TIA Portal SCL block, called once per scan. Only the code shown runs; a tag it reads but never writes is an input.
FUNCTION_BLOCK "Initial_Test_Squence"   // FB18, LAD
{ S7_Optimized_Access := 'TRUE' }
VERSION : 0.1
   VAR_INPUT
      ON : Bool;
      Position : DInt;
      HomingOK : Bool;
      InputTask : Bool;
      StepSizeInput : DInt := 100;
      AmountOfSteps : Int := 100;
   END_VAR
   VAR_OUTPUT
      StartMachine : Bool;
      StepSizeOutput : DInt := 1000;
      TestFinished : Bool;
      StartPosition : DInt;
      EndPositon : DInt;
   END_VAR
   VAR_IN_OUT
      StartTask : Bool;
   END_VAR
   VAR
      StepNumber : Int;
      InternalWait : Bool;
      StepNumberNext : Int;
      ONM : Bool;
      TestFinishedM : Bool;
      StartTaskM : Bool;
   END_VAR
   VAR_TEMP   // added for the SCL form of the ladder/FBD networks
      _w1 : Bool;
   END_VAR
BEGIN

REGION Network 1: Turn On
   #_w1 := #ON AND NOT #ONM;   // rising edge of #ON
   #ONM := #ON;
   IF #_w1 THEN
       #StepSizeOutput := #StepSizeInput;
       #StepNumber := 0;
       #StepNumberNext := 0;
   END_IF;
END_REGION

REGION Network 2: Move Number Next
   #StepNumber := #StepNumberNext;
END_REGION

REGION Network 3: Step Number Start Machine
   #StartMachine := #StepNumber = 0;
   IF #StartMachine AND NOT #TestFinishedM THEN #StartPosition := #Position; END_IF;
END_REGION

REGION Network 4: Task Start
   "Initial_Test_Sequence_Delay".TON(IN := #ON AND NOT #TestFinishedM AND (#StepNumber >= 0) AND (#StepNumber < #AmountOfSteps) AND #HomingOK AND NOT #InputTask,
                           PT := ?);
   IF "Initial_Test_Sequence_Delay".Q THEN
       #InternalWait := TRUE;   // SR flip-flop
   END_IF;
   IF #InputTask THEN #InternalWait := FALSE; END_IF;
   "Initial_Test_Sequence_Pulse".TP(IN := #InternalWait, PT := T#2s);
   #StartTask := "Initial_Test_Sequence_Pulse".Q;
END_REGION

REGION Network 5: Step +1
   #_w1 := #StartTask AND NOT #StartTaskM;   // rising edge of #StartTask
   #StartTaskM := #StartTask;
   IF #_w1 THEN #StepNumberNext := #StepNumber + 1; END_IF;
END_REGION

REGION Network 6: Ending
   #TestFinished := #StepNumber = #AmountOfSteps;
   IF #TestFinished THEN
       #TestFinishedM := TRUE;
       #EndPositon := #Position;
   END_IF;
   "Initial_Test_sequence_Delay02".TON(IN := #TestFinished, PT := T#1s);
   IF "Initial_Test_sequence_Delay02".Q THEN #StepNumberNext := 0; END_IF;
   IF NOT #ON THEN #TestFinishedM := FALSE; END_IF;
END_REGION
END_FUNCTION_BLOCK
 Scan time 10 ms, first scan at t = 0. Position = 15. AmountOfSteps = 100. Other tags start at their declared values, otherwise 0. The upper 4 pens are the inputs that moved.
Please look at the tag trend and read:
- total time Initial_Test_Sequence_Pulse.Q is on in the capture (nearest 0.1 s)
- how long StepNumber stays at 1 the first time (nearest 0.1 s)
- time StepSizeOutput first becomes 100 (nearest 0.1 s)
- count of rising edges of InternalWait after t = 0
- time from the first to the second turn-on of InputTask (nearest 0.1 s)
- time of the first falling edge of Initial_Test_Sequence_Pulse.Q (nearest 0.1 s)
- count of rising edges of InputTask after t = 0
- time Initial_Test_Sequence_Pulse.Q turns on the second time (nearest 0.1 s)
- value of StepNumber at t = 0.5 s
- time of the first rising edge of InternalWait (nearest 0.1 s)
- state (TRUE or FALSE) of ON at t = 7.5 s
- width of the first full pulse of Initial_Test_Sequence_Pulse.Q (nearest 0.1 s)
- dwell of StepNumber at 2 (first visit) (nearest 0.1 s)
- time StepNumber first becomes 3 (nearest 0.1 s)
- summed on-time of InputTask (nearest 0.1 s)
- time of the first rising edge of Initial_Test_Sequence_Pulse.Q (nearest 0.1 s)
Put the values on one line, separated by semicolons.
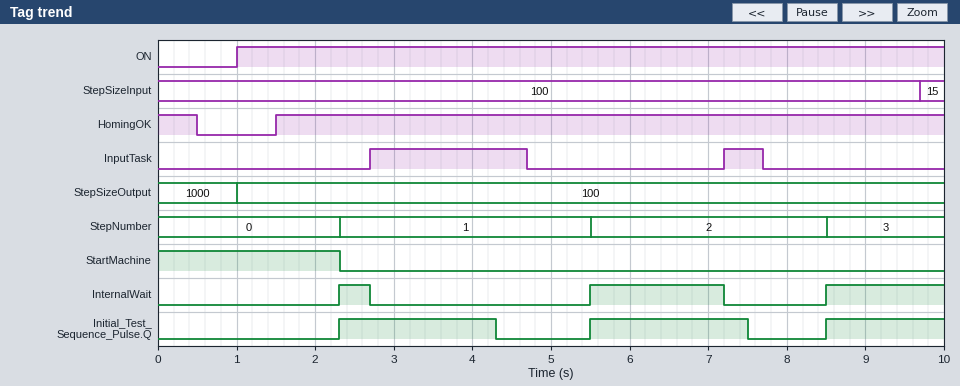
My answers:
5.5 s; 3.2 s; 1.0 s; 3; 4.5 s; 4.3 s; 2; 5.5 s; 0; 2.3 s; TRUE; 2.0 s; 3.0 s; 8.5 s; 2.5 s; 2.3 s
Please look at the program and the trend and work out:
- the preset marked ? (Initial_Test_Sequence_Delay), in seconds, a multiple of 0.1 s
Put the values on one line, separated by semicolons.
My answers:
0.8 s
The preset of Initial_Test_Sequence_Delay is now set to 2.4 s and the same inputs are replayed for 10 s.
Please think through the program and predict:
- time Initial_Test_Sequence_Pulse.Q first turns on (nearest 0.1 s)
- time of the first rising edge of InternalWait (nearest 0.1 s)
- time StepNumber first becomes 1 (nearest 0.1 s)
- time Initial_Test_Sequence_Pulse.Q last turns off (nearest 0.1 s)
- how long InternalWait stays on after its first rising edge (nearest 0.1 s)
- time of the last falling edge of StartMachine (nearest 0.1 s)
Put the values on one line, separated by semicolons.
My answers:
7.1 s; 7.1 s; 7.1 s; 9.1 s; 0.1 s; 7.1 s
